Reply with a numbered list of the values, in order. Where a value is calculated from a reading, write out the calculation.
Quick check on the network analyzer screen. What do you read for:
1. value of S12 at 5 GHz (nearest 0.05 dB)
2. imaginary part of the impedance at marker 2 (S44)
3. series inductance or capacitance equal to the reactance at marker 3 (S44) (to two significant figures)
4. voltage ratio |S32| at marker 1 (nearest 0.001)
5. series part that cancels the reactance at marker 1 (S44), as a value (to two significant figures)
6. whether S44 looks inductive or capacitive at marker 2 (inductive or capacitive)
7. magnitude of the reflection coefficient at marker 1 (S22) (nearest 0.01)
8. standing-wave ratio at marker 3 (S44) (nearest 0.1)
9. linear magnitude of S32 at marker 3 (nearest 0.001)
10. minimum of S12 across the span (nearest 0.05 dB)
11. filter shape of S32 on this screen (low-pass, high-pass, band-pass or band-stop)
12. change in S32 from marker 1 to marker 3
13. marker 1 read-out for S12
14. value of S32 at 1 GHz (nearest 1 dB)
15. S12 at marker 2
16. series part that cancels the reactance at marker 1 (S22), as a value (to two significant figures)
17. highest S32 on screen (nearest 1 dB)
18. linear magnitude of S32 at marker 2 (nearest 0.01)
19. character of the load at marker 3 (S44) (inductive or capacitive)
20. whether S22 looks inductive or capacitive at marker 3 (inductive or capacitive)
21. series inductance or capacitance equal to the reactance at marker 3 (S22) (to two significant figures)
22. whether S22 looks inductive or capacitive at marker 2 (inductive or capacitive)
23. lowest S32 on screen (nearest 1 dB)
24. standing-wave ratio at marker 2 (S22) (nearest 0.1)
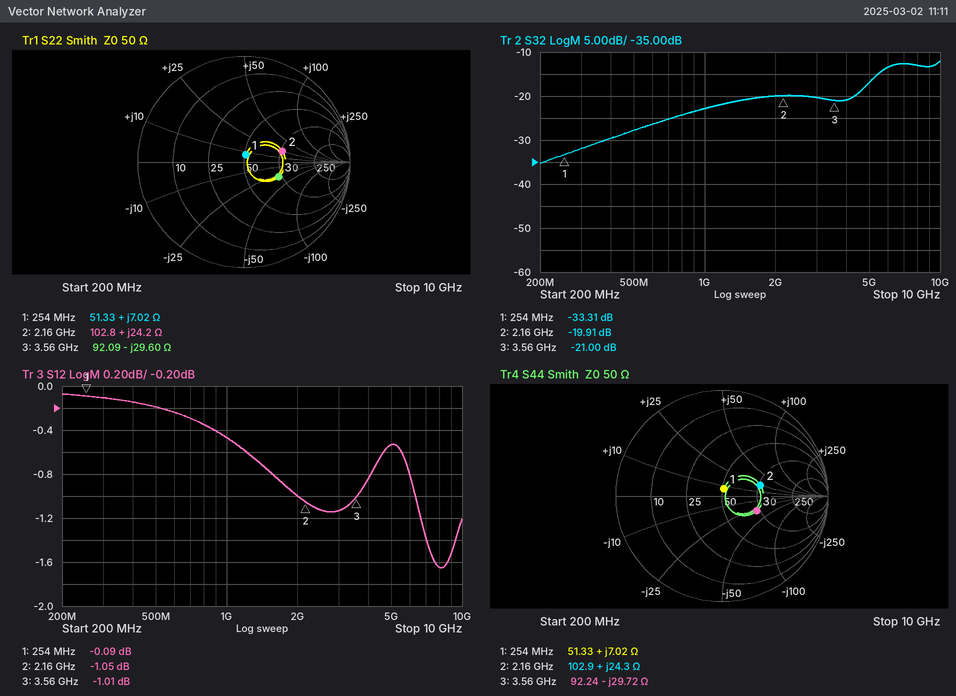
1. -0.55 dB
2. +24.3 Ω
3. C = 1/(2π × 3.56 GHz × 29.72 Ω) ≈ 1.5 pF
4. 10^(-33.31/20) ≈ 0.022
5. C = 1/(2π × 254 MHz × 7.02 Ω) ≈ 89 pF
6. inductive
7. 0.07
8. 2.1
9. 10^(-21/20) ≈ 0.089
10. -1.65 dB
11. high-pass
12. -21 − (-33.31) = 12.31 dB
13. -0.09 dB
14. -23 dB
15. -1.05 dB
16. C = 1/(2π × 254 MHz × 7.02 Ω) ≈ 89 pF
17. -12 dB
18. 10^(-19.91/20) ≈ 0.10
19. capacitive
20. capacitive
21. C = 1/(2π × 3.56 GHz × 29.6 Ω) ≈ 1.5 pF
22. inductive
23. -35 dB
24. 2.2
